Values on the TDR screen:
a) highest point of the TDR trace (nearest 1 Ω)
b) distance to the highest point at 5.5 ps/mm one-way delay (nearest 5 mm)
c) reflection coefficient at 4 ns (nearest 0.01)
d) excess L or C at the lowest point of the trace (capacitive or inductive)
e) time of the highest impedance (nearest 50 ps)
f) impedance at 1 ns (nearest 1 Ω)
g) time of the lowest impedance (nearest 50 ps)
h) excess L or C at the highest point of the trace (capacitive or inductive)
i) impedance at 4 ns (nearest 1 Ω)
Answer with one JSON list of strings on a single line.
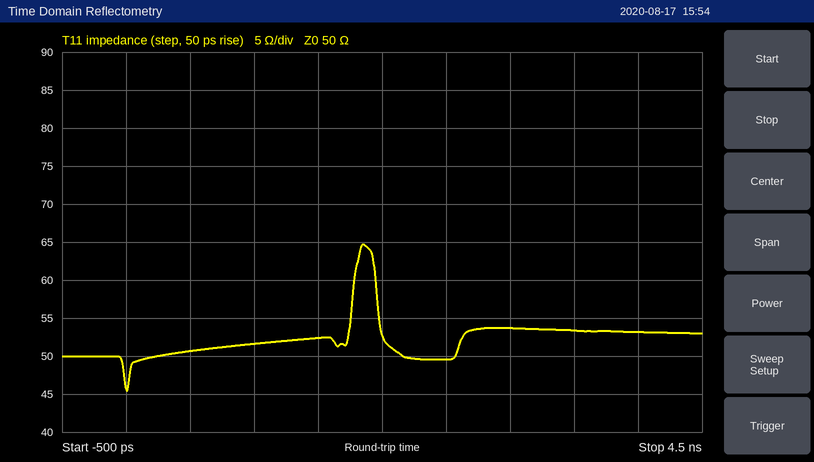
["65 Ω", "170 mm", "+0.03", "capacitive", "1.85 ns", "52 Ω", "0 ps", "inductive", "53 Ω"]
